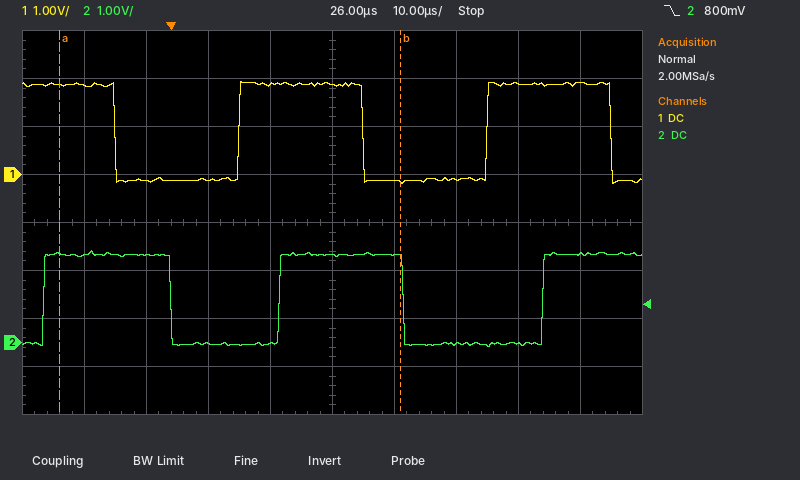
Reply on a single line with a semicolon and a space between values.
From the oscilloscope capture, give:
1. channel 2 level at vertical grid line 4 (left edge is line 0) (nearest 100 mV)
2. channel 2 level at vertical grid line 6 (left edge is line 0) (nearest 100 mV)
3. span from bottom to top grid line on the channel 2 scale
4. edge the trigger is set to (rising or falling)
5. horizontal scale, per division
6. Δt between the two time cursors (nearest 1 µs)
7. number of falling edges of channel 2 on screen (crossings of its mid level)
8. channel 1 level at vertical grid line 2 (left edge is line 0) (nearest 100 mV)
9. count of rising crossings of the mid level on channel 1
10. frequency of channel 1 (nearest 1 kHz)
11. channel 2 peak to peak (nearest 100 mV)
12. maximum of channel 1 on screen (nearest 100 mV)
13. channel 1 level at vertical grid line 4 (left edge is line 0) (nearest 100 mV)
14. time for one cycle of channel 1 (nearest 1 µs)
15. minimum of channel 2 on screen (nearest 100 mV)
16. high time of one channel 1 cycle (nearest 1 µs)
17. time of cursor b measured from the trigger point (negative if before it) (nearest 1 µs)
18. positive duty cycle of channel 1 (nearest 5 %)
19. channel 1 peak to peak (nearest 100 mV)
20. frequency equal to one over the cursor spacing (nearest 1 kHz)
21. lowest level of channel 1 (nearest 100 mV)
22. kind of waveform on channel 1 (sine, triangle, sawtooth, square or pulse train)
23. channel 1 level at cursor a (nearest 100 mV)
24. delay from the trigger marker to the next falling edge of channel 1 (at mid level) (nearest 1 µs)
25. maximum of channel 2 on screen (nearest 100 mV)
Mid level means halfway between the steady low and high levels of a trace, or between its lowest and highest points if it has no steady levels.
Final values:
0.0 V; 1.8 V; 8 V; falling; 10 µs; 55 µs; 2; -100 mV; 2; 25 kHz; 2.0 V; 1.9 V; 1.9 V; 40 µs; -100 mV; 20 µs; +37 µs; 50 %; 2.1 V; 18 kHz; -200 mV; square; 1.9 V; 31 µs; 1.9 V
